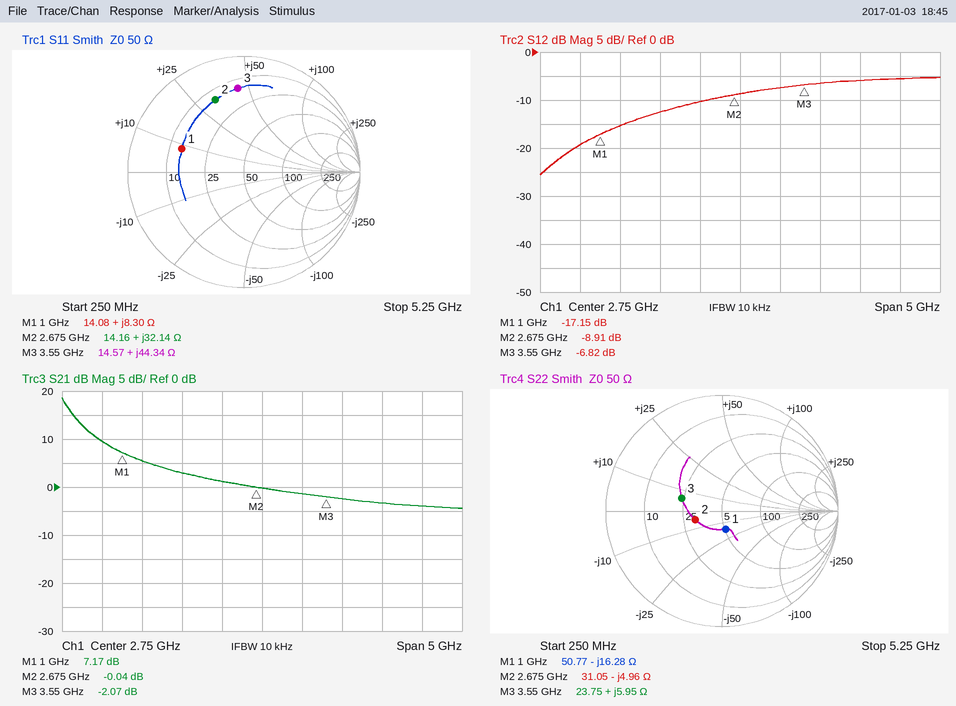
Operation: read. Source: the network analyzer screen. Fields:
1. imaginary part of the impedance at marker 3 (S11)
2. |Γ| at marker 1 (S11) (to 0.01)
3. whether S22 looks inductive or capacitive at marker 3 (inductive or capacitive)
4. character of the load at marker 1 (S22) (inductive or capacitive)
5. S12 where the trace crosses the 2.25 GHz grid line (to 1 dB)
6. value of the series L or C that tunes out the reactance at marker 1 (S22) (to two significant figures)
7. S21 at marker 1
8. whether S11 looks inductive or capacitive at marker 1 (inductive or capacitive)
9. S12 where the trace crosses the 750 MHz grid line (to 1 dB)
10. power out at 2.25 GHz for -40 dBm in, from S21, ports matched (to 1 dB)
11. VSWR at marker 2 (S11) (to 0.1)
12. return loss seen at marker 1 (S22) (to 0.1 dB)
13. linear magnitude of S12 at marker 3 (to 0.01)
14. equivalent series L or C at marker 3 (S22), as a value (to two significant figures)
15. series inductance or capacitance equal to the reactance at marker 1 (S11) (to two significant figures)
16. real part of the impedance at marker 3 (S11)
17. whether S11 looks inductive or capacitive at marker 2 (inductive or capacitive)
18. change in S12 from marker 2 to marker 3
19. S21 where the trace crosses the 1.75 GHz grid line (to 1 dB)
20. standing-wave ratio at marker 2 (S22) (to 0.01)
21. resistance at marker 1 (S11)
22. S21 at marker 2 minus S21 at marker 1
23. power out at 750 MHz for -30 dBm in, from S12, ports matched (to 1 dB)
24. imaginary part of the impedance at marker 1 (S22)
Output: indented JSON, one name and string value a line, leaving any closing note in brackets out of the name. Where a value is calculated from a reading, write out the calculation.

{
  "imaginary part of the impedance at marker 3": "+44.34 Ω",
  "|Γ| at marker 1 (S11)": "0.57",
  "whether S22 looks inductive or capacitive at marker 3": "inductive",
  "character of the load at marker 1 (S22)": "capacitive",
  "S12 where the trace crosses the 2.25 GHz grid line": "-10 dB",
  "value of the series L or C that tunes out the reactance at marker 1 (S22)": "L = 16.28 Ω/(2π × 1 GHz) ≈ 2.6 nH",
  "S21 at marker 1": "7.17 dB",
  "whether S11 looks inductive or capacitive at marker 1": "inductive",
  "S12 where the trace crosses the 750 MHz grid line": "-19 dB",
  "power out at 2.25 GHz for -40 dBm in, from S21, ports matched": "-40 dBm + (1 dB) = -39 dBm",
  "VSWR at marker 2 (S11)": "5.1",
  "return loss seen at marker 1 (S22)": "15.9 dB",
  "linear magnitude of S12 at marker 3": "10^(-6.82/20) ≈ 0.46",
  "equivalent series L or C at marker 3 (S22), as a value": "L = 5.95 Ω/(2π × 3.55 GHz) ≈ 267 pH, so 270 pH to two significant figures",
  "series inductance or capacitance equal to the reactance at marker 1 (S11)": "L = 8.3 Ω/(2π × 1 GHz) ≈ 1.3 nH",
  "real part of the impedance at marker 3": "14.57 Ω",
  "whether S11 looks inductive or capacitive at marker 2": "inductive",
  "change in S12 from marker 2 to marker 3": "-6.82 − (-8.91) = 2.09 dB",
  "S21 where the trace crosses the 1.75 GHz grid line": "3 dB",
  "standing-wave ratio at marker 2 (S22)": "1.64",
  "resistance at marker 1": "14.08 Ω",
  "S21 at marker 2 minus S21 at marker 1": "-0.04 − (7.17) = -7.21 dB",
  "power out at 750 MHz for -30 dBm in, from S12, ports matched": "-30 dBm + (-19 dB) = -49 dBm",
  "imaginary part of the impedance at marker 1": "-16.28 Ω"
}
